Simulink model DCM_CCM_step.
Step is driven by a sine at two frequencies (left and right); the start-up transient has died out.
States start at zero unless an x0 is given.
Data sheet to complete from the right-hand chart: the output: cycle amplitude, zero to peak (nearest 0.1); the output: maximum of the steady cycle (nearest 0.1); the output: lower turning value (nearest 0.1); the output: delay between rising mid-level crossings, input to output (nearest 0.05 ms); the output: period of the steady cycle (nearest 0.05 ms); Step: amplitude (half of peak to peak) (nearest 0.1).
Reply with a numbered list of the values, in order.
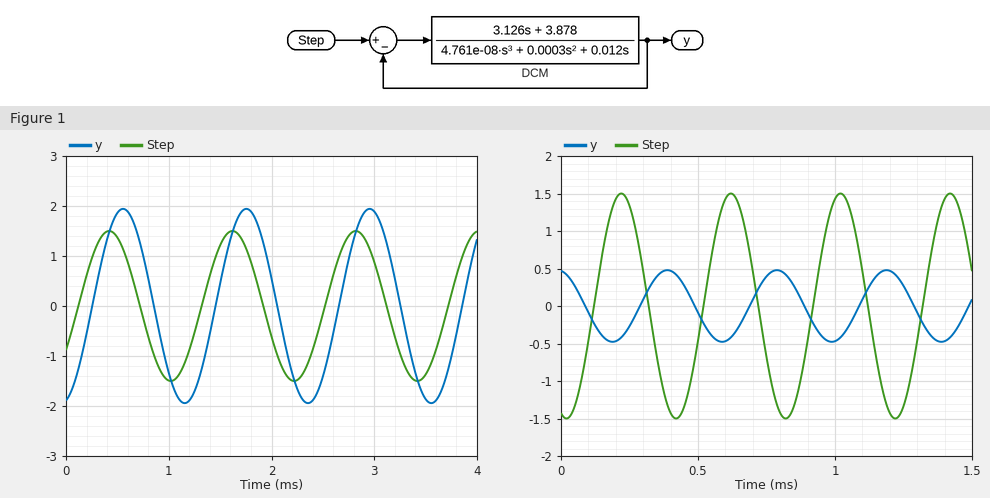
1. 0.5
2. 0.5
3. -0.5
4. 0.15 ms
5. 0.40 ms
6. 1.5
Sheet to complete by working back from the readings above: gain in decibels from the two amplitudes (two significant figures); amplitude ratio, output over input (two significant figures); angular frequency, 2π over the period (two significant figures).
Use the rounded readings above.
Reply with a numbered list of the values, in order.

1. -9.5 dB
2. 0.33
3. 16 rad/ms
